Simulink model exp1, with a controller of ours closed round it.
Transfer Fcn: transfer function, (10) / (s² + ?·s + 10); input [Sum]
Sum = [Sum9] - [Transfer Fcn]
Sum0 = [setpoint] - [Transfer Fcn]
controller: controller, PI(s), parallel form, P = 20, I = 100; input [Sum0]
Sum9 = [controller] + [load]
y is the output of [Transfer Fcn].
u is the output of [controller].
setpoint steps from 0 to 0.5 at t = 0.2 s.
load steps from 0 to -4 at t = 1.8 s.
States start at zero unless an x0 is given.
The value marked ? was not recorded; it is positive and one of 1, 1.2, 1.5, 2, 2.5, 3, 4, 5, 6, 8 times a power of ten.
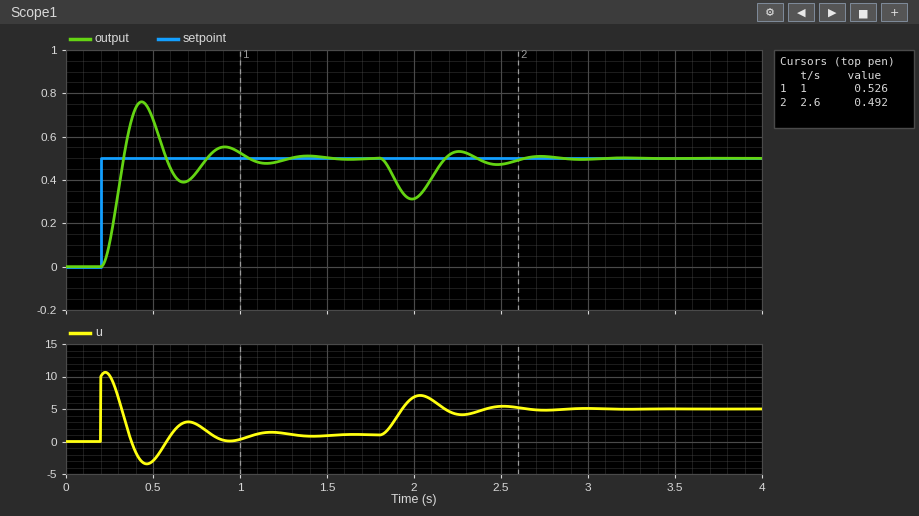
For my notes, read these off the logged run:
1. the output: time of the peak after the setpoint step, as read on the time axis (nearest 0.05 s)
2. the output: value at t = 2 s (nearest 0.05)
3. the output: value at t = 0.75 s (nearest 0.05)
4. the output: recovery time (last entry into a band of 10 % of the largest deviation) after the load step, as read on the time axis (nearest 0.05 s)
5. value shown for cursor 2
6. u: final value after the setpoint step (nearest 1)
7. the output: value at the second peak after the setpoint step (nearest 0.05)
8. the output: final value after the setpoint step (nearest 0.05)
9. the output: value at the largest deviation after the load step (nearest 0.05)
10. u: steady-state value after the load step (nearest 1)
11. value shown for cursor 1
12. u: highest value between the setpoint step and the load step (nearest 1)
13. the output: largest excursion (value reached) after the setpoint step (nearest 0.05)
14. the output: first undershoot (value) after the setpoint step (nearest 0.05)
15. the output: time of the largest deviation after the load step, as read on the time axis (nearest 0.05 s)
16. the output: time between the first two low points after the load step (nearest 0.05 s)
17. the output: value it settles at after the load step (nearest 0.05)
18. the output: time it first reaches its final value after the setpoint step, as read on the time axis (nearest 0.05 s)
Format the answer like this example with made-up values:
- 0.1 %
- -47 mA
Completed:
- 0.45 s
- 0.30
- 0.45
- 2.55 s
- 0.492
- 1
- 0.55
- 0.50
- 0.30
- 5
- 0.526
- 11
- 0.75
- 0.40
- 2.00 s
- 0.50 s
- 0.50
- 0.35 s
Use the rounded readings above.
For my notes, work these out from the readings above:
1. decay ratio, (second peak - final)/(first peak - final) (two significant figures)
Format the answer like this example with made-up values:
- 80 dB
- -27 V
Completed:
- 0.20
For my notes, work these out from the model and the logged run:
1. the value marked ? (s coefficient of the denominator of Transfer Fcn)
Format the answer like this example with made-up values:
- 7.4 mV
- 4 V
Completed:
- 12
